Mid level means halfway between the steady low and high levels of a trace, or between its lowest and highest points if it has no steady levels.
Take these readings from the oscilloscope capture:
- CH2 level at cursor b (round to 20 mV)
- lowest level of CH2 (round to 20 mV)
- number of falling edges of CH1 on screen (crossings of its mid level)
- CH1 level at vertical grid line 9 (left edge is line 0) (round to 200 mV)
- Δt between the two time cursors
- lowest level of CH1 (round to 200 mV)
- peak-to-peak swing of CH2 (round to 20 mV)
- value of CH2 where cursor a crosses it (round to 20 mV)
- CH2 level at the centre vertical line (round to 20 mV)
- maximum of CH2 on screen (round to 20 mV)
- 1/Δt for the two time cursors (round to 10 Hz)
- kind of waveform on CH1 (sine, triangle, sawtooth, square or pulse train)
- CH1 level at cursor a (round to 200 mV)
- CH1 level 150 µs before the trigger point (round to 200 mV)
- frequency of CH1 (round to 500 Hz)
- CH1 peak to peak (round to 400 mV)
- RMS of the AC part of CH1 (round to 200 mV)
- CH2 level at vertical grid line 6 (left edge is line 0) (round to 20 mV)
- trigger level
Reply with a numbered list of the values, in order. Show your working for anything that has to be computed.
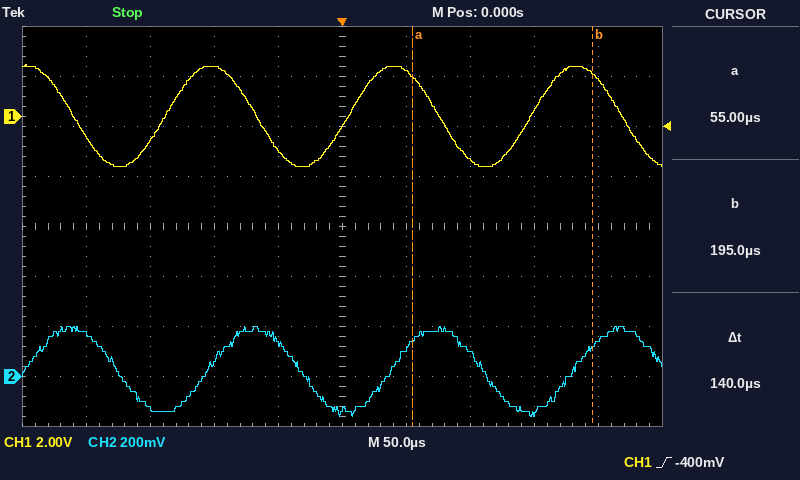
1. 120 mV
2. -160 mV
3. 4
4. 1.4 V
5. 140 µs
6. -2.0 V
7. 200 mV − (-160 mV) = 360 mV
8. 140 mV
9. -140 mV
10. 200 mV
11. 1 / 140 µs ≈ 7.14 kHz
12. sine
13. 1.6 V
14. -1.0 V
15. 7.0 kHz
16. 4.0 V
17. 4.0 V / (2√2) ≈ 1.4 V
18. 120 mV
19. -400 mV
